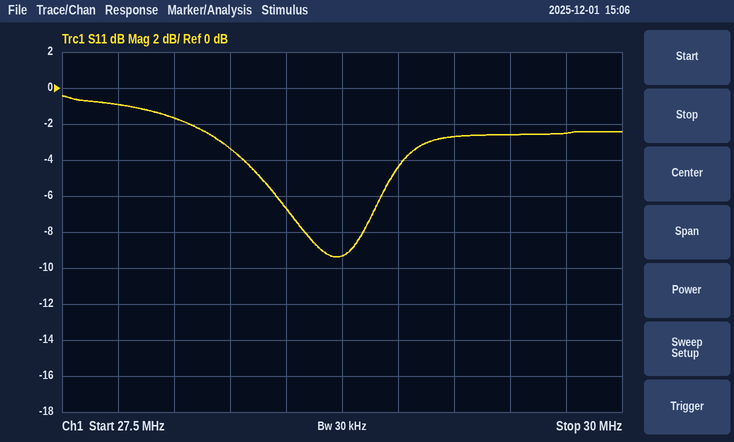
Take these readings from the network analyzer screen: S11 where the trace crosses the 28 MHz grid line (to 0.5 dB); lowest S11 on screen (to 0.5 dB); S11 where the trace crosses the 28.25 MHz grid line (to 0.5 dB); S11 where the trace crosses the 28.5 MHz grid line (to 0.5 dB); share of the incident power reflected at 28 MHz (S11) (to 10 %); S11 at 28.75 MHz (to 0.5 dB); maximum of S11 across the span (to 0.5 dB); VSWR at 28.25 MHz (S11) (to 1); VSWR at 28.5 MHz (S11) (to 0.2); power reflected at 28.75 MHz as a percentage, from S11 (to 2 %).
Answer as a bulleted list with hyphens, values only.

- -1.5 dB
- -9.5 dB
- -3.5 dB
- -6.5 dB
- 70 %
- -9.5 dB
- -0.5 dB
- 5
- 2.8
- 12 %
